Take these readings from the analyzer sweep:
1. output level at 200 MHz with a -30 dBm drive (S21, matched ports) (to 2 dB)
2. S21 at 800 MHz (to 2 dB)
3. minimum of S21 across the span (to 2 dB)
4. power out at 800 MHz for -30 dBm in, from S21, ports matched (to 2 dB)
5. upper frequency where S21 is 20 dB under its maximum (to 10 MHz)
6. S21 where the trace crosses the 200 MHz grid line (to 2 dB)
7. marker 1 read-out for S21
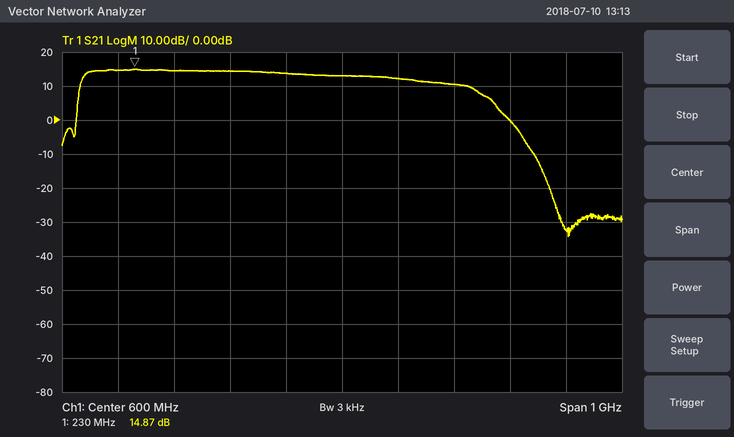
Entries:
-16 dBm
10 dB
-34 dB
-20 dBm
920 MHz
14 dB
14.87 dB
